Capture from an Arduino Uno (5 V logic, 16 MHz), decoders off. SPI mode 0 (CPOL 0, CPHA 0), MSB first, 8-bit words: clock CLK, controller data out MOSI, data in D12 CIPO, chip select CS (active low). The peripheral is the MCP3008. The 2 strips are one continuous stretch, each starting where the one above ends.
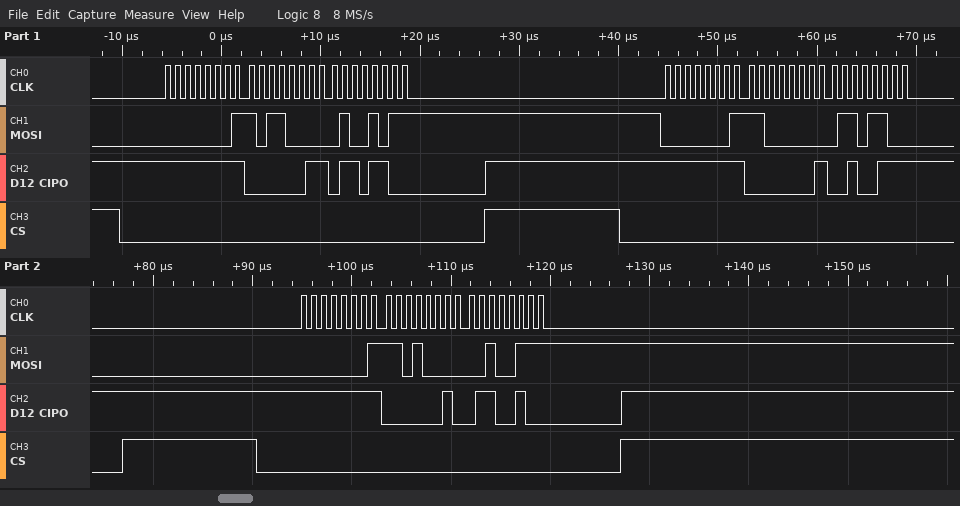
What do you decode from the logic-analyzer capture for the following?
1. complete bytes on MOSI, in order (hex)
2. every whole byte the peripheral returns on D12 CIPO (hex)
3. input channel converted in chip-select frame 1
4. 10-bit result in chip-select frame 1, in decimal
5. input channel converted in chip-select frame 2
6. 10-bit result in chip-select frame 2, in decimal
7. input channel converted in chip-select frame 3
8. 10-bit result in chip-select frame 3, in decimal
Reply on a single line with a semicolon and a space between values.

01 B0 4B 01 C0 6C 01 D0 27; FF 03 6C FF 01 27 FF 02 64; 3; 876; 4; 295; 5; 612
